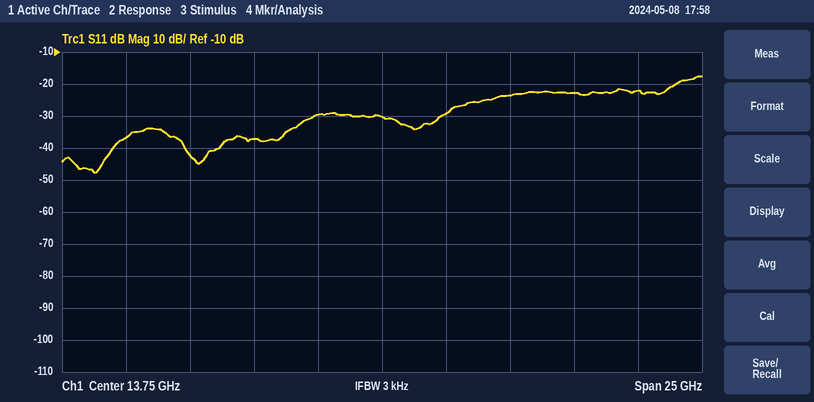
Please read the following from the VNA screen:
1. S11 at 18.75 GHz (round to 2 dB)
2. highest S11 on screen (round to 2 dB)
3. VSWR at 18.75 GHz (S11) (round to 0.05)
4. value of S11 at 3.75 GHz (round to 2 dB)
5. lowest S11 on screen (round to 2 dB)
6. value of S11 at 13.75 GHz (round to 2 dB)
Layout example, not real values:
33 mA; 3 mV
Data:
-24 dB; -18 dB; 1.15; -36 dB; -48 dB; -30 dB
